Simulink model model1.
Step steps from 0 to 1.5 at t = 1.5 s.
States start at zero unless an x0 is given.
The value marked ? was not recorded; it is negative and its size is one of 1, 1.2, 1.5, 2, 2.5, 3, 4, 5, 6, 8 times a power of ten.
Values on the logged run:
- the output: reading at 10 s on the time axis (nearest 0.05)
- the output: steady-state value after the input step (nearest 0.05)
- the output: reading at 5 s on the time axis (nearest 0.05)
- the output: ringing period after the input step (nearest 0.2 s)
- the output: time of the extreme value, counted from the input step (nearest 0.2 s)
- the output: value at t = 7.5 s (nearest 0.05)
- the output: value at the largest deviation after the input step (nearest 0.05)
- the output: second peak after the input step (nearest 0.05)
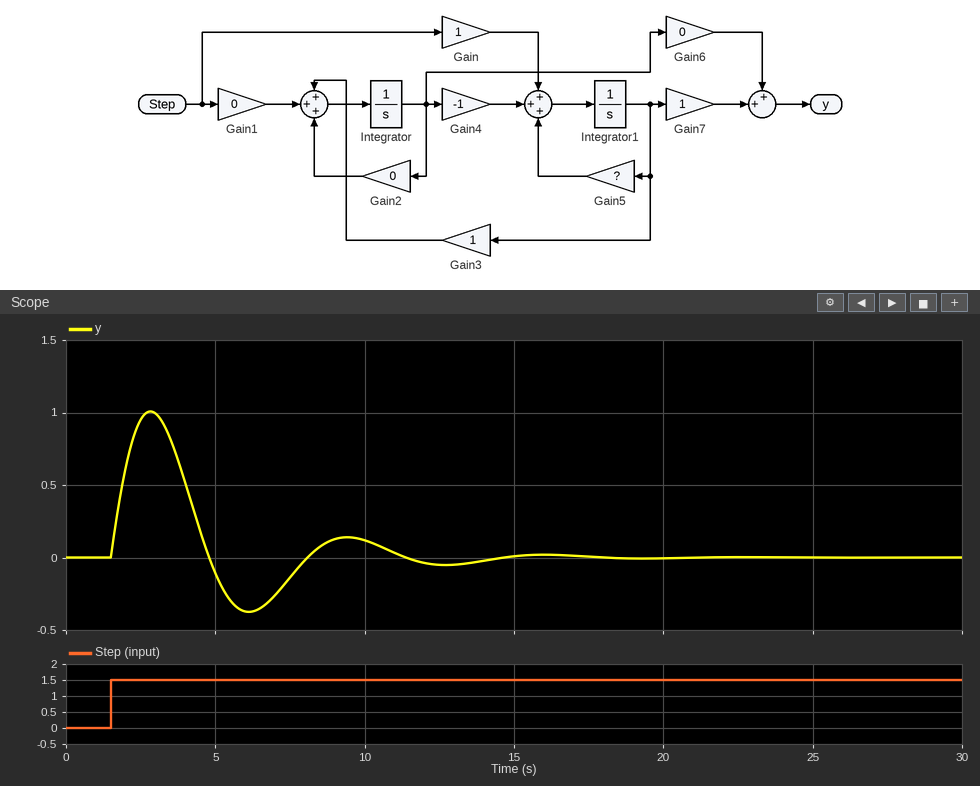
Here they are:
0.10
0.00
-0.10
6.6 s
1.4 s
-0.15
1.00
0.15
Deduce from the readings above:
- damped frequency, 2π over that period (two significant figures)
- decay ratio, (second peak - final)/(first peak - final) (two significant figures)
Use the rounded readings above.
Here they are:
0.95 rad/s
0.15
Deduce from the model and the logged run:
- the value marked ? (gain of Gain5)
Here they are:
-0.6
